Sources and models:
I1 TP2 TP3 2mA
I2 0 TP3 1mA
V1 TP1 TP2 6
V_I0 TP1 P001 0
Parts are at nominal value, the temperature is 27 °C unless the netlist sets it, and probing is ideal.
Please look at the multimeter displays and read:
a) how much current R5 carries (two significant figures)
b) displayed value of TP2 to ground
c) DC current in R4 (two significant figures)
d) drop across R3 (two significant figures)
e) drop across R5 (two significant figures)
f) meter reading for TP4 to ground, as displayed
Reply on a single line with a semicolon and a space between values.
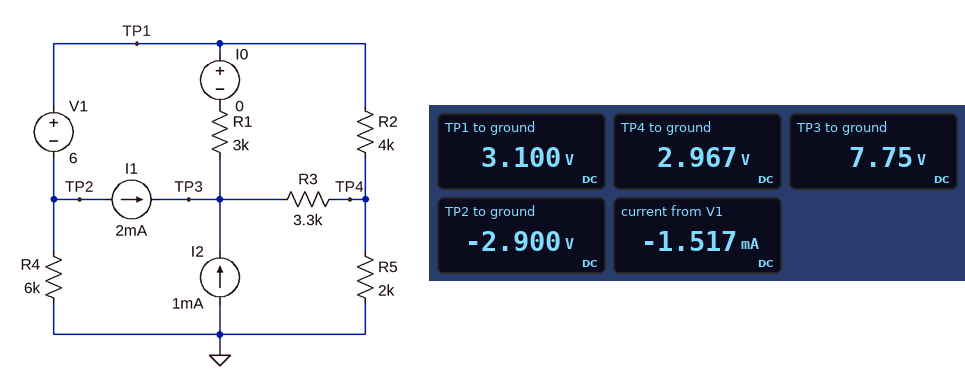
1.5 mA; -2.900 V; 480 µA; 4.8 V; 3.0 V; 2.967 V
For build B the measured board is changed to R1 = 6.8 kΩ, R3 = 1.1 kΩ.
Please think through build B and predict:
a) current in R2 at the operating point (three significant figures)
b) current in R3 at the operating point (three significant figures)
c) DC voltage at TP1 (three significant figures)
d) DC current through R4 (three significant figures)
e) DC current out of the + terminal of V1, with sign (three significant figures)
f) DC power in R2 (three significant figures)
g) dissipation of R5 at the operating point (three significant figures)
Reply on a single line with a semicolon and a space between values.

539 µA; 2.31 mA; 1.38 V; 770 µA; -1.23 mA; 1.16 mW; 6.26 mW
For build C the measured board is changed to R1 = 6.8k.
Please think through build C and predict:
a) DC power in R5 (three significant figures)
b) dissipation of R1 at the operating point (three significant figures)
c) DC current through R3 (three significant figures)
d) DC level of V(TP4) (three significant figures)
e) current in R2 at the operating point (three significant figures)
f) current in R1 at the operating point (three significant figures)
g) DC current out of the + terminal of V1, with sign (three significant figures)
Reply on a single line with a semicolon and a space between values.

5.36 mW; 8.06 mW; 1.91 mA; 3.27 V; 274 µA; 1.09 mA; -1.36 mA
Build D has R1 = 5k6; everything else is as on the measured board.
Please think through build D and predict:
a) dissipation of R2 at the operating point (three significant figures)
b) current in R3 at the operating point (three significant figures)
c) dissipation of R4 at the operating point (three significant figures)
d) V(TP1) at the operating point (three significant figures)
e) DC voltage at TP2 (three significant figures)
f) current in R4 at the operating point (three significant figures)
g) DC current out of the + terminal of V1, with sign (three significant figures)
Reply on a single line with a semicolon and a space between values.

158 µW; 1.80 mA; 2.16 mW; 2.40 V; -3.60 V; 599 µA; -1.40 mA
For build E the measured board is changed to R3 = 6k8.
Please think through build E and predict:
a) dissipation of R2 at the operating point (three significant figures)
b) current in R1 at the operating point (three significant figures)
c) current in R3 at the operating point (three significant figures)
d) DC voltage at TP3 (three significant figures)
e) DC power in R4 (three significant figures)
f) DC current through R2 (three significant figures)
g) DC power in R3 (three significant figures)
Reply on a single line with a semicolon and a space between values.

372 µW; 1.96 mA; 1.04 mA; 9.79 V; 725 µW; 305 µA; 7.39 mW
